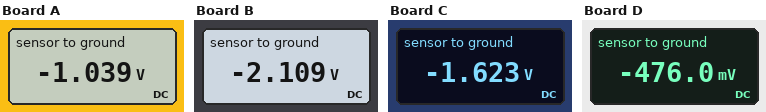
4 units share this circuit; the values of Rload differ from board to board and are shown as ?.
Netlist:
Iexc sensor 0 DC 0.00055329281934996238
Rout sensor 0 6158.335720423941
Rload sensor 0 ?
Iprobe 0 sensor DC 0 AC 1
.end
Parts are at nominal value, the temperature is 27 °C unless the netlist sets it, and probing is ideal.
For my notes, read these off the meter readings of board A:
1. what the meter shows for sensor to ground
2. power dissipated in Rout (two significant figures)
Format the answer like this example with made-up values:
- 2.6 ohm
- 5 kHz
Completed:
- -1.039 V
- 180 µW
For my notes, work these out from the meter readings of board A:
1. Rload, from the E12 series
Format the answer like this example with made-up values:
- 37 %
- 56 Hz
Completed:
- 2.7 kΩ
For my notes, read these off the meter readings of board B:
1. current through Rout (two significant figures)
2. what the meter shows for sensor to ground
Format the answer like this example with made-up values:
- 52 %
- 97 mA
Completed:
- 340 µA
- -2.109 V
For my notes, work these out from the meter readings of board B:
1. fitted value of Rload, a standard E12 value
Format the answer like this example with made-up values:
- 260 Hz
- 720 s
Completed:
- 10 kΩ
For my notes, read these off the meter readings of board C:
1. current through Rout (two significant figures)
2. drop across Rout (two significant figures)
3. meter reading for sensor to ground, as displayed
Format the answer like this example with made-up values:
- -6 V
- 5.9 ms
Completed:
- 260 µA
- 1.6 V
- -1.623 V
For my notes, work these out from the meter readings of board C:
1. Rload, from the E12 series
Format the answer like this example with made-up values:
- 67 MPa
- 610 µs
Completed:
- 5.6 kΩ
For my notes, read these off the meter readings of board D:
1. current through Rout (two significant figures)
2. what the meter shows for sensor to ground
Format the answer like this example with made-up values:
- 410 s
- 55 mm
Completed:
- 77 µA
- -476.0 mV
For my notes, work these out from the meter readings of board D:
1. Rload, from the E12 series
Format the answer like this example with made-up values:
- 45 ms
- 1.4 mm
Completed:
- 1 kΩ
